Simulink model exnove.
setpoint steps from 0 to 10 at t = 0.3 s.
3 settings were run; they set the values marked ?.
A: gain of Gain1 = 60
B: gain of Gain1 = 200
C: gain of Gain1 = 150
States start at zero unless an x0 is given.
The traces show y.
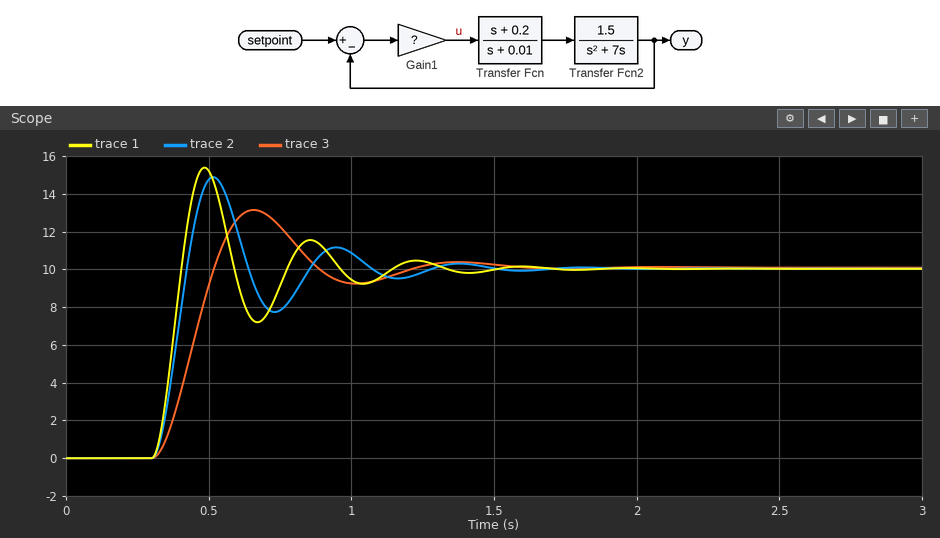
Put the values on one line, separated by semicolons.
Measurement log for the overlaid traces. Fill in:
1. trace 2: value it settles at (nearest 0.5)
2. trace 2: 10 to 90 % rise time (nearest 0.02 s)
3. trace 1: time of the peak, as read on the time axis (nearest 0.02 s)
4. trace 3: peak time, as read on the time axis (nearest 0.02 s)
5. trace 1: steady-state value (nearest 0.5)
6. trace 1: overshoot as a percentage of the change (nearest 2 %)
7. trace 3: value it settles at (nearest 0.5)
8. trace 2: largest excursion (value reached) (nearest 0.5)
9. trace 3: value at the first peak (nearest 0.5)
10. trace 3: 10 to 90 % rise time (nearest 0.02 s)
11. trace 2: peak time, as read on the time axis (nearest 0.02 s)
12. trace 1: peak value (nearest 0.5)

10.0; 0.08 s; 0.48 s; 0.66 s; 10.0; 54 %; 10.0; 15.0; 13.0; 0.14 s; 0.52 s; 15.5
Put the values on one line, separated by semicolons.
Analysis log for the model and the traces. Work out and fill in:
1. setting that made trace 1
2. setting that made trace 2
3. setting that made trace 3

B; C; A
